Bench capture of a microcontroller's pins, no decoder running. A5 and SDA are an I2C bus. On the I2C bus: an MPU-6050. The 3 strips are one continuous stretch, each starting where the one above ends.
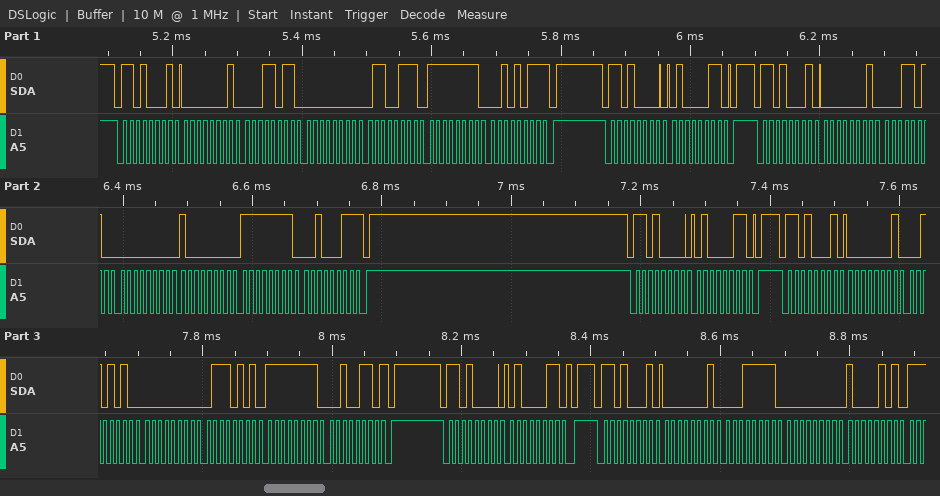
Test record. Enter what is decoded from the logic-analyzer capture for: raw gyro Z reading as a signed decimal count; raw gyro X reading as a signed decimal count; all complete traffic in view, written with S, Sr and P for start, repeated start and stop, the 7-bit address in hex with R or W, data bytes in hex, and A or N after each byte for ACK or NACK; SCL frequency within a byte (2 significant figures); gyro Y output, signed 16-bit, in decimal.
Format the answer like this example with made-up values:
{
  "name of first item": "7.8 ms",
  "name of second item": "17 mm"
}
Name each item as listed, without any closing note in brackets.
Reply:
{
  "raw gyro Z reading as a signed decimal count": "-221",
  "raw gyro X reading as a signed decimal count": "282",
  "all complete traffic in view, written with S, Sr and P for start, repeated start and stop, the 7-bit address in hex with R or W, data bytes in hex, and A or N after each byte for ACK or NACK": "S 68R A 01 A 1B A 00 A 67 A FF A 2B N P S 68W A 43 A P S 68R A 01 A 1A A 00 A 80 A FF A 23 N P S 68W A 43 A P S 68R A 01 A 2A A 00 A 75 A FF A 26 N P S 68W A 43 A P S 68R A 01 A 1F A 00 A 85 A",
  "SCL frequency within a byte": "100 kHz",
  "gyro Y output, signed 16-bit, in decimal": "128"
}
